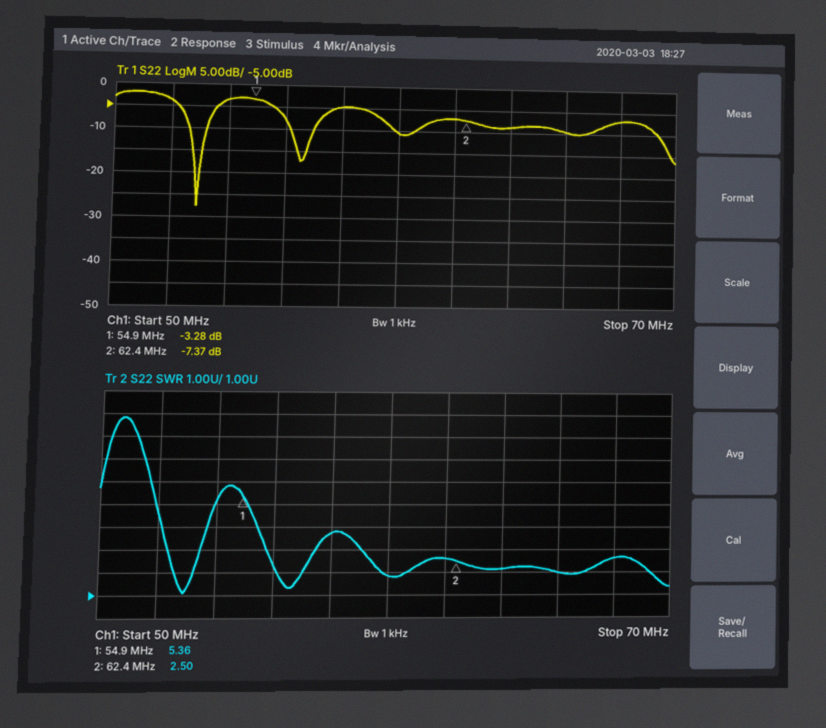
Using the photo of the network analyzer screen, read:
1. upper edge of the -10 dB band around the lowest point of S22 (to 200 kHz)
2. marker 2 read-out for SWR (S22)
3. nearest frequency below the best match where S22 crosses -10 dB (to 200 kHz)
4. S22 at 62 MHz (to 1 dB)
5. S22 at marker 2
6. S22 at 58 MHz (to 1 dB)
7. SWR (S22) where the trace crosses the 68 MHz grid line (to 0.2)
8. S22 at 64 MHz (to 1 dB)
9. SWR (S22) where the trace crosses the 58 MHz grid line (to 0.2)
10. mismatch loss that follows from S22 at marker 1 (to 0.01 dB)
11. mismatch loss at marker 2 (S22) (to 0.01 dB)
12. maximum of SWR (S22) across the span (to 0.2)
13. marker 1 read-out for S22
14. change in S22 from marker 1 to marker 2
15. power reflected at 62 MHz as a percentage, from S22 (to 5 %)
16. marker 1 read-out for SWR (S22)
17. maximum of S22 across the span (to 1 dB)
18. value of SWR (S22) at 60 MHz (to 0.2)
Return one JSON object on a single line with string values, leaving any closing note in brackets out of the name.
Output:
{"upper edge of the -10 dB band around the lowest point of S22": "53.2 MHz", "marker 2 read-out for SWR": "2.50", "nearest frequency below the best match where S22 crosses -10 dB": "52.6 MHz", "S22 at 62 MHz": "-7 dB", "S22 at marker 2": "-7.37 dB", "S22 at 58 MHz": "-5 dB", "SWR (S22) where the trace crosses the 68 MHz grid line": "2.6", "S22 at 64 MHz": "-9 dB", "SWR (S22) where the trace crosses the 58 MHz grid line": "3.8", "mismatch loss that follows from S22 at marker 1": "2.76 dB", "mismatch loss at marker 2 (S22)": "0.88 dB", "maximum of SWR (S22) across the span": "8.8", "marker 1 read-out for S22": "-3.28 dB", "change in S22 from marker 1 to marker 2": "-4.09 dB", "power reflected at 62 MHz as a percentage, from S22": "20 %", "marker 1 read-out for SWR": "5.36", "maximum of S22 across the span": "-2 dB", "value of SWR (S22) at 60 MHz": "1.8"}
